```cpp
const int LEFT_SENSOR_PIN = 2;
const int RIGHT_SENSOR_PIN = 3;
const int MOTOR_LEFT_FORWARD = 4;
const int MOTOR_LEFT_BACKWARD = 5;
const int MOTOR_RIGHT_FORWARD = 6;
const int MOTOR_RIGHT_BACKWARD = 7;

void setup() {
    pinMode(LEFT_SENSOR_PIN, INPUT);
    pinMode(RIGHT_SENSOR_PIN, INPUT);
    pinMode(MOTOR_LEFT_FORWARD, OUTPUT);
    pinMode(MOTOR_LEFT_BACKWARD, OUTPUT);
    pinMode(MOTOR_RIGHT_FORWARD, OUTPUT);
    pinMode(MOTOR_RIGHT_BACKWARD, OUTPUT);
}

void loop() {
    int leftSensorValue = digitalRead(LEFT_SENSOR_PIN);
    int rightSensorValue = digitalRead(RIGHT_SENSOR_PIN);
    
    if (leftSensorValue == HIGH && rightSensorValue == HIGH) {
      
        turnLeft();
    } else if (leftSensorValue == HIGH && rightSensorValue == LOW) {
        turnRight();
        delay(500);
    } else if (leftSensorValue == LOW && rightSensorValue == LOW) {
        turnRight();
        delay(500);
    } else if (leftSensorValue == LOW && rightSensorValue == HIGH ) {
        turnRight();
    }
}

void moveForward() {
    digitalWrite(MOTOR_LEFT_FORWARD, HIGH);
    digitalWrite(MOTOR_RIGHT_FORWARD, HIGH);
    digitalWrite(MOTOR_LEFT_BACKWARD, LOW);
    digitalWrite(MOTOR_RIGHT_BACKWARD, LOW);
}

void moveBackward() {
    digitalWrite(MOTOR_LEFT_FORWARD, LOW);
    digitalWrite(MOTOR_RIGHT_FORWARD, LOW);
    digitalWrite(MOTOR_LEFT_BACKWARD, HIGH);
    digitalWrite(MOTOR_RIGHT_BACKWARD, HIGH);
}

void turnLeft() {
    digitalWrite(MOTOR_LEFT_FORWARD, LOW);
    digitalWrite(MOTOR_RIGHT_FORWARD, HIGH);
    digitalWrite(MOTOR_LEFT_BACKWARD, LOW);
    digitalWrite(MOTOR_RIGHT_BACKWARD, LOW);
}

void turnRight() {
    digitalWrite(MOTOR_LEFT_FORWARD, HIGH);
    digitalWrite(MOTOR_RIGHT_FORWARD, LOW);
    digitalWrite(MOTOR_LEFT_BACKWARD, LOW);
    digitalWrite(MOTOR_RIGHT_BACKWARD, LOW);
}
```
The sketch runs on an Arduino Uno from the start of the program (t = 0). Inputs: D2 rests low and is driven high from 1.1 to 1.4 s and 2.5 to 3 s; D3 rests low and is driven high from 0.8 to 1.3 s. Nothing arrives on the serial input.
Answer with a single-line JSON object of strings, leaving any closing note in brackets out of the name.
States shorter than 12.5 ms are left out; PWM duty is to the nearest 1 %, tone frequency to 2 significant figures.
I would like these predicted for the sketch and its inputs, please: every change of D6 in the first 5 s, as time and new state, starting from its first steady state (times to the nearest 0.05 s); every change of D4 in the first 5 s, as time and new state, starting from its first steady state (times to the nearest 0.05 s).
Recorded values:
{"every change of D6 in the first 5 s, as time and new state, starting from its first steady state": "0 s low; 1.1 s high; 1.3 s low", "every change of D4 in the first 5 s, as time and new state, starting from its first steady state": "0 s high; 1.1 s low; 1.3 s high"}
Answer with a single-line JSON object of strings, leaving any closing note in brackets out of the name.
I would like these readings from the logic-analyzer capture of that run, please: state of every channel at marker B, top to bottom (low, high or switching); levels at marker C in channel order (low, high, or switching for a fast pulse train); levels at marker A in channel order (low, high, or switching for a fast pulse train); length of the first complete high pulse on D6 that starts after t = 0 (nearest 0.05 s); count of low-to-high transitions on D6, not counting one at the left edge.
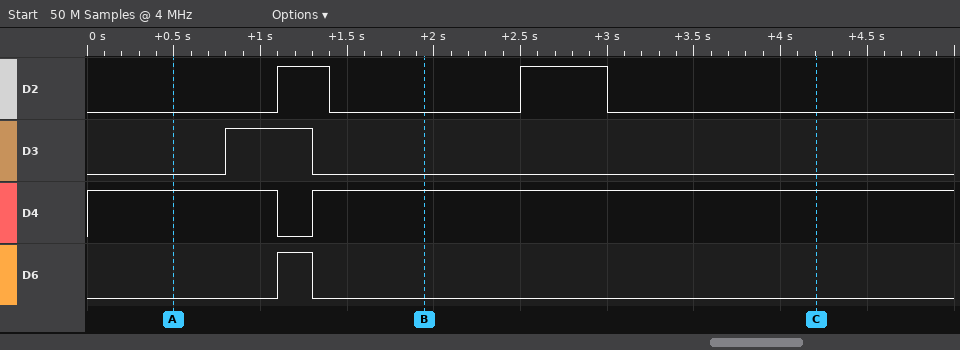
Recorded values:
{"state of every channel at marker B, top to bottom": "D2 low, D3 low, D4 high, D6 low", "levels at marker C in channel order": "D2 low, D3 low, D4 high, D6 low", "levels at marker A in channel order": "D2 low, D3 low, D4 high, D6 low", "length of the first complete high pulse on D6 that starts after t = 0": "0.20 s", "count of low-to-high transitions on D6, not counting one at the left edge": "1"}
